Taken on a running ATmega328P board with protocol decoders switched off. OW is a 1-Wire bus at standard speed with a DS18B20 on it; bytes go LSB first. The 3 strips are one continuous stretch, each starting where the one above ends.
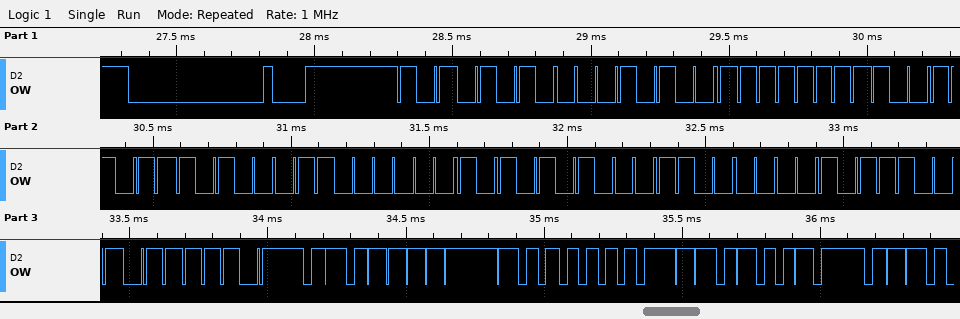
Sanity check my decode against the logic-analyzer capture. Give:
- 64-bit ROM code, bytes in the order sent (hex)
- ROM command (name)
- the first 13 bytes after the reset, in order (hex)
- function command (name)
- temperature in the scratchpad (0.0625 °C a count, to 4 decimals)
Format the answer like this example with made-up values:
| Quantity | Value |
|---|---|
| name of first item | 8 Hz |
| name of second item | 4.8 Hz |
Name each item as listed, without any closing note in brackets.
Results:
| Quantity | Value |
|---|---|
| 64-bit ROM code, bytes in the order sent | 28 FF D9 C5 40 15 03 9D |
| ROM command | Match ROM |
| the first 13 bytes after the reset, in order | 55 28 FF D9 C5 40 15 03 9D BE FA 01 4B |
| function command | Read Scratchpad |
| temperature in the scratchpad | 31.6250 °C |
